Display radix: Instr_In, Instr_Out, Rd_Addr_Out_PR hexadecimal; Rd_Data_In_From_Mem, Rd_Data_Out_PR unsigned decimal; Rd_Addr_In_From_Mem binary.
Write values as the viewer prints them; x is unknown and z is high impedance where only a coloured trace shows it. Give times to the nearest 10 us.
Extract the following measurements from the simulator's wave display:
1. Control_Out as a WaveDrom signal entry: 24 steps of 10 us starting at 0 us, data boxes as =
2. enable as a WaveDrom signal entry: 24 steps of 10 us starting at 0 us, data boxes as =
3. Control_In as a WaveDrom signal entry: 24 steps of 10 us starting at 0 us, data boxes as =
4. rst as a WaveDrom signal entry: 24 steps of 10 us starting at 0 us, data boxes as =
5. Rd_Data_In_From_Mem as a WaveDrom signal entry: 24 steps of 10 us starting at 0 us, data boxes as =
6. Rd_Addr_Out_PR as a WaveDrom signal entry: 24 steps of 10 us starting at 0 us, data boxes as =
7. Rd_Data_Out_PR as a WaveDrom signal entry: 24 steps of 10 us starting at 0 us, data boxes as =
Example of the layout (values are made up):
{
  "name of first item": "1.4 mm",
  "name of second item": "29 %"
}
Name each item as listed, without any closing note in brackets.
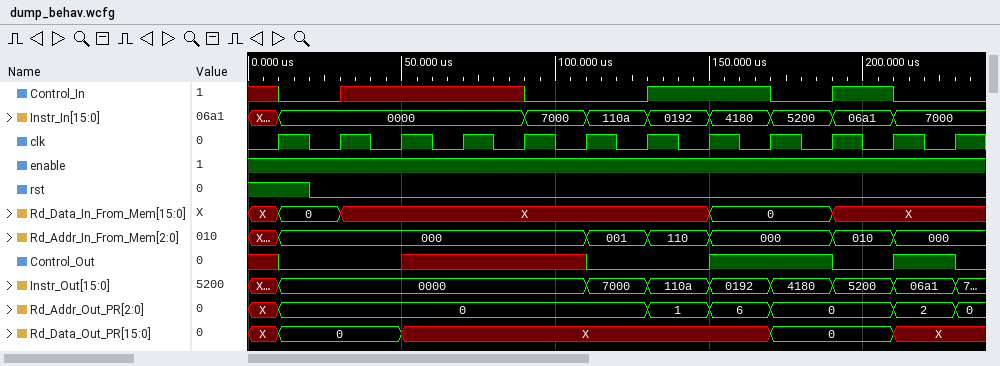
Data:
{
  "Control_Out as a WaveDrom signal entry: 24 steps of 10 us starting at 0 us, data boxes as =": "{name: 'Control_Out', wave: 'x0...x.....0...1...0.1.0'}",
  "enable as a WaveDrom signal entry: 24 steps of 10 us starting at 0 us, data boxes as =": "{name: 'enable', wave: '1.......................'}",
  "Control_In as a WaveDrom signal entry: 24 steps of 10 us starting at 0 us, data boxes as =": "{name: 'Control_In', wave: 'x0.x.....0...1...0.1.0..'}",
  "rst as a WaveDrom signal entry: 24 steps of 10 us starting at 0 us, data boxes as =": "{name: 'rst', wave: '1.0.....................'}",
  "Rd_Data_In_From_Mem as a WaveDrom signal entry: 24 steps of 10 us starting at 0 us, data boxes as =": "{name: 'Rd_Data_In_From_Mem', wave: 'x=.x...........=...x....', data: '0 0'}",
  "Rd_Addr_Out_PR as a WaveDrom signal entry: 24 steps of 10 us starting at 0 us, data boxes as =": "{name: 'Rd_Addr_Out_PR', wave: 'x=...........=.=.=...=.=', data: '0 1 6 0 2 0'}",
  "Rd_Data_Out_PR as a WaveDrom signal entry: 24 steps of 10 us starting at 0 us, data boxes as =": "{name: 'Rd_Data_Out_PR', wave: 'x=...x...........=...x..', data: '0 0'}"
}
